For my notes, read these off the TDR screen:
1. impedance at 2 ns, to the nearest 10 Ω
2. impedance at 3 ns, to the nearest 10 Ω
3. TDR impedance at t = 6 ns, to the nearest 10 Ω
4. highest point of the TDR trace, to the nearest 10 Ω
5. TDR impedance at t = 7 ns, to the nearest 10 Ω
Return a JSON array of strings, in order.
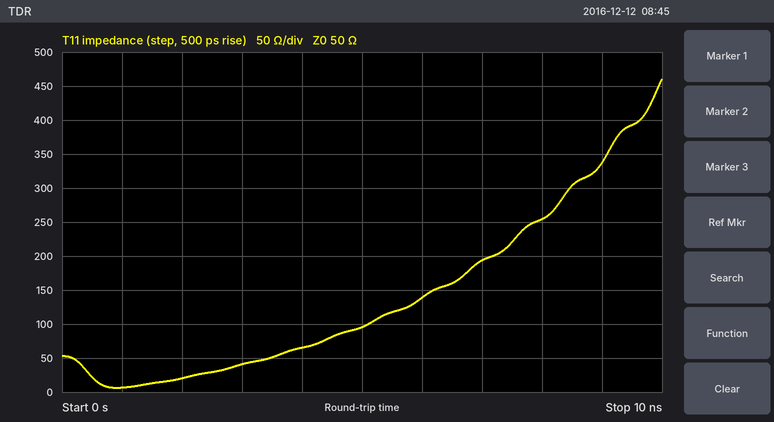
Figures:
["20 Ω", "40 Ω", "140 Ω", "460 Ω", "190 Ω"]
